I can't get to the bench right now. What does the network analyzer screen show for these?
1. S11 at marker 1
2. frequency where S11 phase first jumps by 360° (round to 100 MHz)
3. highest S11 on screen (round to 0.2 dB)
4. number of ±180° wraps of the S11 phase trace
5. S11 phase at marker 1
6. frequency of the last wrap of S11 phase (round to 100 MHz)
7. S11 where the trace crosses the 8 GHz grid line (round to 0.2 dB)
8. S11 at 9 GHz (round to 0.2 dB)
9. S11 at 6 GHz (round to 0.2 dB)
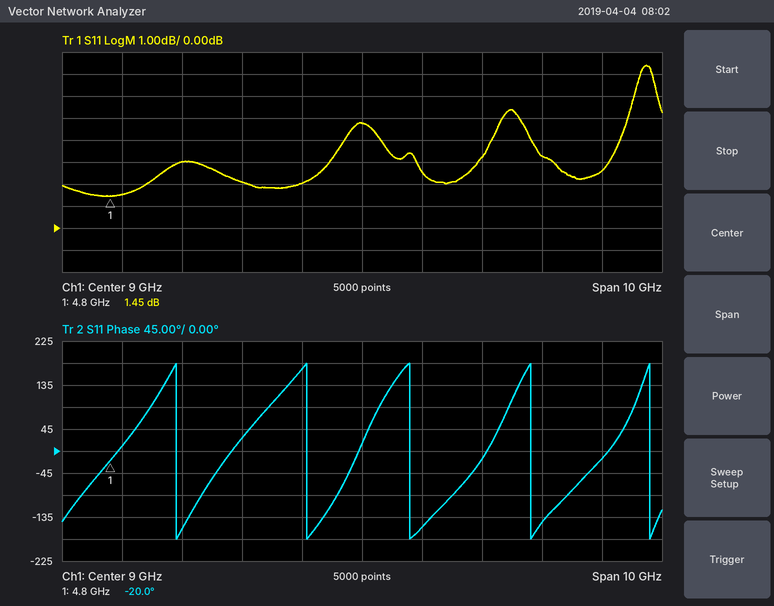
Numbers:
1.45 dB
5.9 GHz
7.4 dB
5
-20.0°
13.8 GHz
2.0 dB
4.8 dB
3.0 dB
